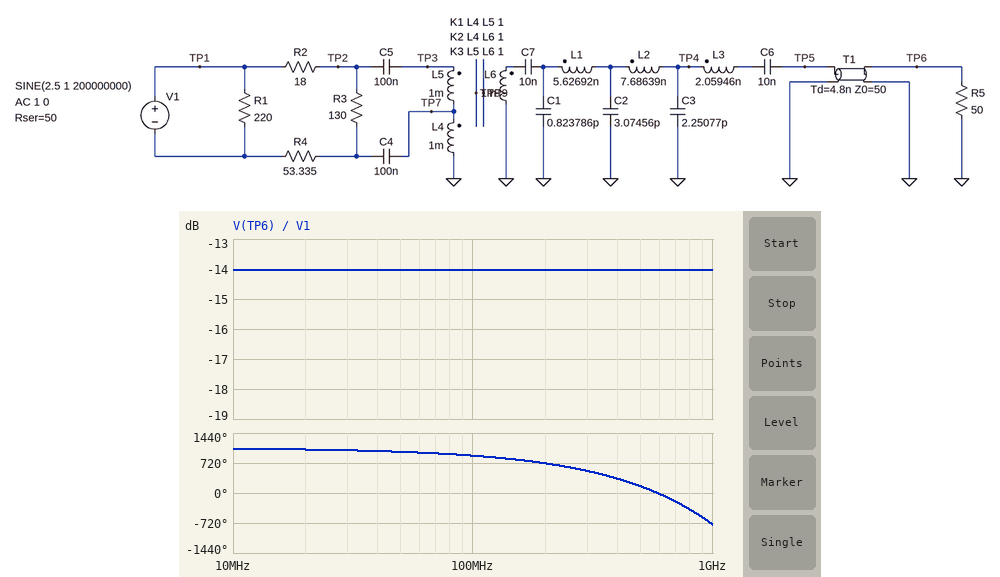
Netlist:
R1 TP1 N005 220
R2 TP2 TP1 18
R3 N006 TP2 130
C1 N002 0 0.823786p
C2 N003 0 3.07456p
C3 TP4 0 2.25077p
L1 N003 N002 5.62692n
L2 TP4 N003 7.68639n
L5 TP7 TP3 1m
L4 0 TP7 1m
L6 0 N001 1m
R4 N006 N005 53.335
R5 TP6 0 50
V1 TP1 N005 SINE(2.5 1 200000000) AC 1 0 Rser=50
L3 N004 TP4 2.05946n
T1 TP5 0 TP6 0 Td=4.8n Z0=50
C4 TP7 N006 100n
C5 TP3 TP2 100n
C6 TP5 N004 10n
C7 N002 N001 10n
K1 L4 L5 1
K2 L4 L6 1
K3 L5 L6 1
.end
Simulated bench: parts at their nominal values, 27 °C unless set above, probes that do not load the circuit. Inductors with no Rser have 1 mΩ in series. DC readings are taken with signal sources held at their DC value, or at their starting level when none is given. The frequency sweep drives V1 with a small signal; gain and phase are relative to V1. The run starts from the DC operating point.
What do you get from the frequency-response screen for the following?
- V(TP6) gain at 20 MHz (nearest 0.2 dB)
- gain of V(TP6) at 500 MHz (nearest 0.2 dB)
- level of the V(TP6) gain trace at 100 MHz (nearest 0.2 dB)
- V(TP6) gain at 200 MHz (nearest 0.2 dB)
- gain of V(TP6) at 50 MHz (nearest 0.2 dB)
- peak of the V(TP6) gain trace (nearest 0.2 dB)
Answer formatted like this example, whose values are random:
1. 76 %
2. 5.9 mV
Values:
1. -14.0 dB
2. -14.0 dB
3. -14.0 dB
4. -14.0 dB
5. -14.0 dB
6. -14.0 dB
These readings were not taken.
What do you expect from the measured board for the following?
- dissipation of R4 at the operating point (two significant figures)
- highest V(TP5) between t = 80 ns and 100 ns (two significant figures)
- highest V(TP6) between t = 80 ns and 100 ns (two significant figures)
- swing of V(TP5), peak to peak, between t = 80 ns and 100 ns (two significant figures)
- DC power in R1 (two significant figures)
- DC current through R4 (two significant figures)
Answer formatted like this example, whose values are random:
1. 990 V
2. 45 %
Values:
1. 3.8 mW
2. 200 mV
3. 200 mV
4. 400 mV
5. 13 mW
6. 8.4 mA
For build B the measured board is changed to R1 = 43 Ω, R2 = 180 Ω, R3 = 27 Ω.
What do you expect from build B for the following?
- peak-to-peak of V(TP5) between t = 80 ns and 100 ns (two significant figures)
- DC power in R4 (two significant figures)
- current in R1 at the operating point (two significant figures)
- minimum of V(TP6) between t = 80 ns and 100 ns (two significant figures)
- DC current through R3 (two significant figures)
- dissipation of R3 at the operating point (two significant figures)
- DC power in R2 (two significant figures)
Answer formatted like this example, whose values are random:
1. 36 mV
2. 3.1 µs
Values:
1. 59 mV
2. 890 µW
3. 25 mA
4. -30 mV
5. 4.1 mA
6. 450 µW
7. 3.0 mW
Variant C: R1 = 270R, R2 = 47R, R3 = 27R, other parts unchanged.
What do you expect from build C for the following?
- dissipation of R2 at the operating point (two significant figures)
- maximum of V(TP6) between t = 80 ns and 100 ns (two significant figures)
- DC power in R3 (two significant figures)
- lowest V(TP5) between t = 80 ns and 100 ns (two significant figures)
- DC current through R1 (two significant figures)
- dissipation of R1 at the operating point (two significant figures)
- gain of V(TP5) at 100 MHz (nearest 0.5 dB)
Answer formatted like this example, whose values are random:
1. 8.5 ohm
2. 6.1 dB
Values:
1. 7.3 mW
2. 92 mV
3. 4.2 mW
4. -93 mV
5. 5.9 mA
6. 9.3 mW
7. -20.5 dB
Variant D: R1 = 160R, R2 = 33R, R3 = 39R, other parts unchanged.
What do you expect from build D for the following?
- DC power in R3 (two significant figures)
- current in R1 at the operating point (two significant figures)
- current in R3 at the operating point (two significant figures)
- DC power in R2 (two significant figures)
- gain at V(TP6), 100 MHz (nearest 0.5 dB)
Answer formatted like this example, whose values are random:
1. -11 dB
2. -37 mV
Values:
1. 5.3 mW
2. 9.1 mA
3. 12 mA
4. 4.5 mW
5. -19.0 dB
